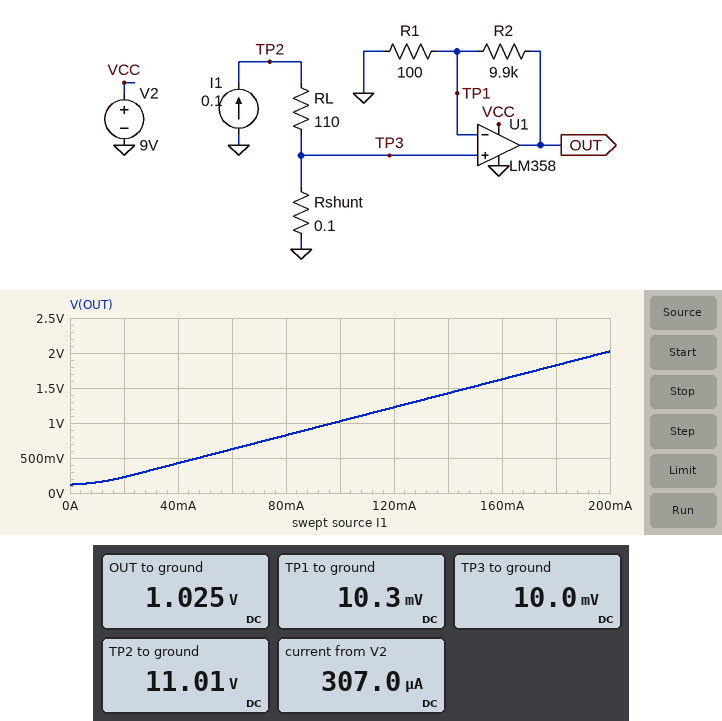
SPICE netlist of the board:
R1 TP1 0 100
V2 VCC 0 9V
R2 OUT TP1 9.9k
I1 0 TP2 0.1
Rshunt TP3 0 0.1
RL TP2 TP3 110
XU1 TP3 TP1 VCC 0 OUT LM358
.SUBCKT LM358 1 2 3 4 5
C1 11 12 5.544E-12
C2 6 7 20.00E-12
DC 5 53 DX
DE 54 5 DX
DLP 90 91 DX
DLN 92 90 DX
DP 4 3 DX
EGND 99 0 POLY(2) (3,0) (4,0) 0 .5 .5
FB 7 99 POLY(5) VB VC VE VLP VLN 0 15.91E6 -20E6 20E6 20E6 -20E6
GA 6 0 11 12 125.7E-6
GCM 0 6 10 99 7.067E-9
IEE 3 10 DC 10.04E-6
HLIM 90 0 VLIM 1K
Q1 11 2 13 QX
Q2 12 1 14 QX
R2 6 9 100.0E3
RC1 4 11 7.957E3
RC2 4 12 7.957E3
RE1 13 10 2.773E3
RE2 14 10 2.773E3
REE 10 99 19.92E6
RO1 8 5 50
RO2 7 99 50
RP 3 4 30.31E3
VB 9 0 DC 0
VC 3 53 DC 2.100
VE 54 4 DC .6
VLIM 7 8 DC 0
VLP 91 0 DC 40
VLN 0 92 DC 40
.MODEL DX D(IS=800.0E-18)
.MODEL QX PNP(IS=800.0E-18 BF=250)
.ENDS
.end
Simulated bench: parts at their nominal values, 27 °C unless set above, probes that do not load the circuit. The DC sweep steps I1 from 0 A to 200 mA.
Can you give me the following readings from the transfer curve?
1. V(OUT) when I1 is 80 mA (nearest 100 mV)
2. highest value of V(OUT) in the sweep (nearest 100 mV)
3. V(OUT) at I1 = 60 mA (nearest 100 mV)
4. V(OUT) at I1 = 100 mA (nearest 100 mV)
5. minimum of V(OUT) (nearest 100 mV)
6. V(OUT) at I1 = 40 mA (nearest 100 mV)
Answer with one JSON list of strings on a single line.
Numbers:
["800 mV", "2.0 V", "600 mV", "1.0 V", "100 mV", "400 mV"]
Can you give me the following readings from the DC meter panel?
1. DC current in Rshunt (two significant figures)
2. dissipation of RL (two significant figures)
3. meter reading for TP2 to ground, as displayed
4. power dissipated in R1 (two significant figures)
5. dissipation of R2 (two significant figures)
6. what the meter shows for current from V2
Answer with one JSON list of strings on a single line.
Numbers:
["100 mA", "1.1 W", "11.01 V", "1.1 µW", "100 µW", "307.0 µA"]
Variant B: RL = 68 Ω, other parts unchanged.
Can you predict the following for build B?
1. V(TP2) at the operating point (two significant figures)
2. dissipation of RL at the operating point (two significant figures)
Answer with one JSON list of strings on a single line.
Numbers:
["6.8 V", "680 mW"]
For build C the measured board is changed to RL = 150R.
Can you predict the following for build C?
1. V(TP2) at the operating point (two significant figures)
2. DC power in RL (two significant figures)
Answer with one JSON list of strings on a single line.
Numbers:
["15 V", "1.5 W"]
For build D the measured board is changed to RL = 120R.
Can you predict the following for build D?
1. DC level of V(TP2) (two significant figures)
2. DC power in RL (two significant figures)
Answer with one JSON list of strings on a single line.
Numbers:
["12 V", "1.2 W"]
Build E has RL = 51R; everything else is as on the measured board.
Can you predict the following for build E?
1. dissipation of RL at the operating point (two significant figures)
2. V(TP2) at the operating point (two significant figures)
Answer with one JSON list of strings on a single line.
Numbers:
["510 mW", "5.1 V"]
